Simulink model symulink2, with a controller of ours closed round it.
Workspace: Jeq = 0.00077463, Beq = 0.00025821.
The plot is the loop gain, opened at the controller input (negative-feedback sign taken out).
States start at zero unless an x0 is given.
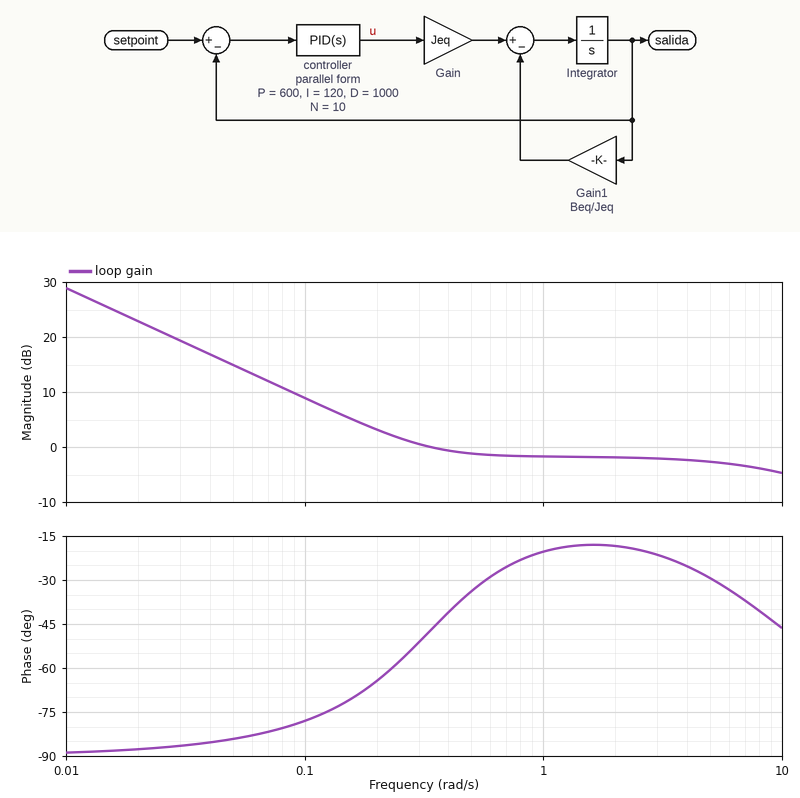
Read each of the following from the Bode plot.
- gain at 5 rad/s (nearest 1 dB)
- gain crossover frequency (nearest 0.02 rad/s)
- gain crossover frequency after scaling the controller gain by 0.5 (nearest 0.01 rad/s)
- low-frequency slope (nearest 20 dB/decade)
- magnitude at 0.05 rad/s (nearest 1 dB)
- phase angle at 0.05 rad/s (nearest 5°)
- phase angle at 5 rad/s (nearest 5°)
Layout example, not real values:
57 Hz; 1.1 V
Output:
-3 dB; 0.34 rad/s; 0.14 rad/s; -20 dB/decade; 15 dB; -85°; -30°
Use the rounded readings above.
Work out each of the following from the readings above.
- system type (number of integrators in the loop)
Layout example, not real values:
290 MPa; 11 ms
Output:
1
